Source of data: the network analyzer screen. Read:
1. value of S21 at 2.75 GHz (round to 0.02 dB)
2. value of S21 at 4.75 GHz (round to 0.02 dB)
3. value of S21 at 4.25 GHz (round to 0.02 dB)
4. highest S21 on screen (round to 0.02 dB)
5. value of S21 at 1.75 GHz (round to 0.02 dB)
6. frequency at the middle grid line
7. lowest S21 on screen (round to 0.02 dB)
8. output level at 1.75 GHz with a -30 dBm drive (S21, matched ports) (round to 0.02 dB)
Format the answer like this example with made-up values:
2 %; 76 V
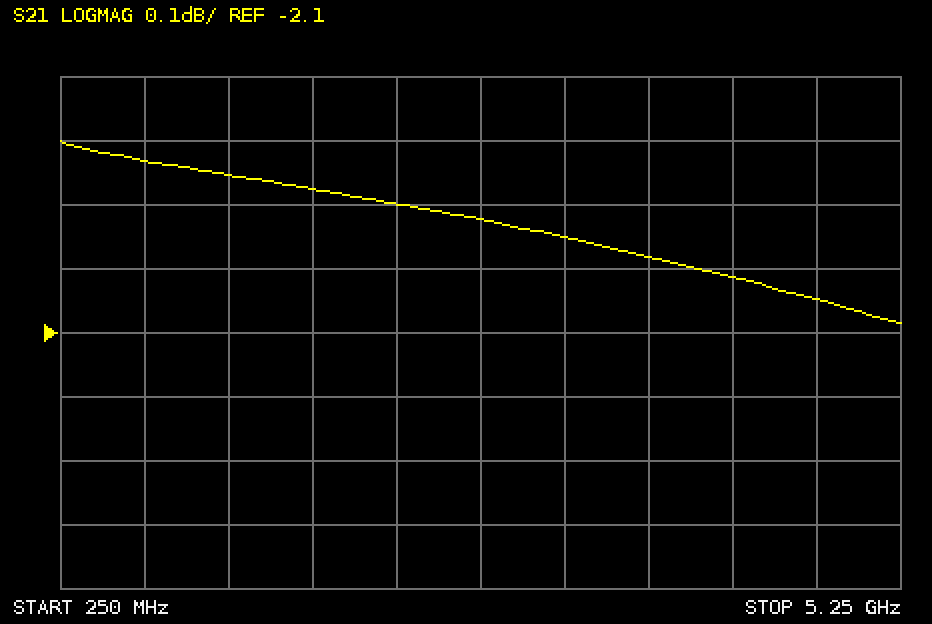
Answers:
-1.92 dB; -2.04 dB; -2.02 dB; -1.80 dB; -1.88 dB; 2.75 GHz; -2.08 dB; -31.88 dBm
